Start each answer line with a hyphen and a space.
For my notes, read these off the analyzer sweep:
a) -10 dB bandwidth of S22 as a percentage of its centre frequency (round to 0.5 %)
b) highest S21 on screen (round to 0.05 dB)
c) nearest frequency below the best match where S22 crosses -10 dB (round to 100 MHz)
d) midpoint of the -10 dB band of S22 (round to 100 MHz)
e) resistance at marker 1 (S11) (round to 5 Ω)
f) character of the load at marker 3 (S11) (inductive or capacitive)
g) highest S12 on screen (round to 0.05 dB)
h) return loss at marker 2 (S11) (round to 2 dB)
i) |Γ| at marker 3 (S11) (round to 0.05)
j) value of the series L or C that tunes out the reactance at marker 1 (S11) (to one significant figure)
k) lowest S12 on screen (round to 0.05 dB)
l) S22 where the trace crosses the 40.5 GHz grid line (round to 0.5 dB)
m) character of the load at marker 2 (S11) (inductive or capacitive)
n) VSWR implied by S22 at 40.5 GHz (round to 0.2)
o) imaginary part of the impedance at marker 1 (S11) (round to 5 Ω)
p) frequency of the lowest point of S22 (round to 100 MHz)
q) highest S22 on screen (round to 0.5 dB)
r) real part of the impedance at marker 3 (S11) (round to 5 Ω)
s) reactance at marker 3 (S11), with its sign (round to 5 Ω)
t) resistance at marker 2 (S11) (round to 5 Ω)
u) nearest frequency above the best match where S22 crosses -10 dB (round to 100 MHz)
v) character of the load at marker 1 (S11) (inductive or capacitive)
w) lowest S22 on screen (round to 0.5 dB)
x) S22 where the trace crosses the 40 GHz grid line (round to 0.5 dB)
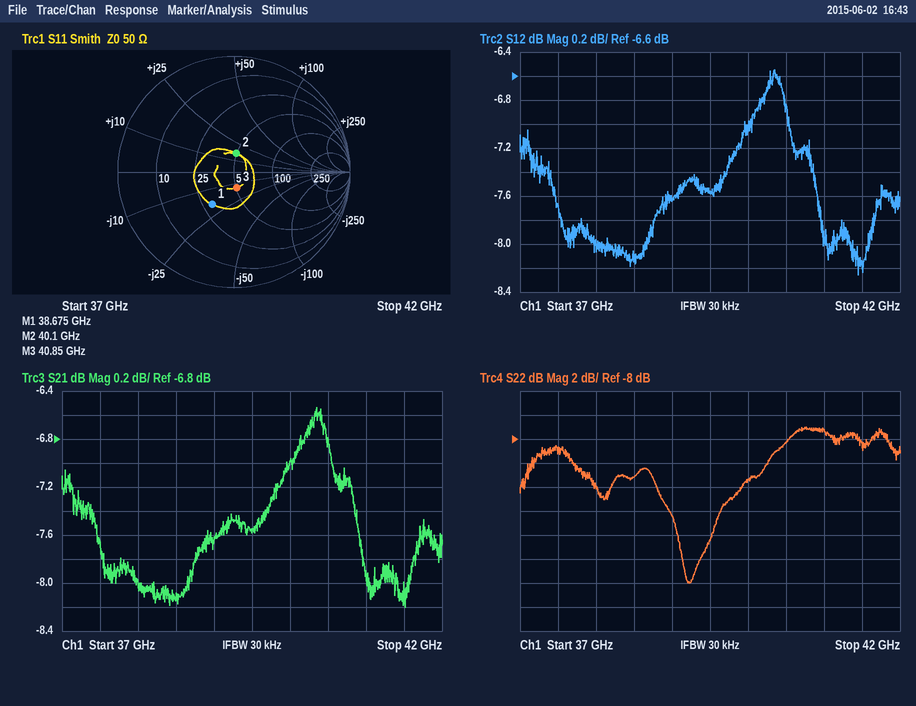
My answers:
- 6.5 %
- -6.55 dB
- 37.7 GHz
- 39.0 GHz
- 30 Ω
- capacitive
- -6.55 dB
- 16 dB
- 0.15
- 80 pH
- -8.25 dB
- -8.5 dB
- inductive
- 2.2
- -20 Ω
- 39.2 GHz
- -7.0 dB
- 50 Ω
- -15 Ω
- 50 Ω
- 40.3 GHz
- capacitive
- -20.0 dB
- -11.5 dB
